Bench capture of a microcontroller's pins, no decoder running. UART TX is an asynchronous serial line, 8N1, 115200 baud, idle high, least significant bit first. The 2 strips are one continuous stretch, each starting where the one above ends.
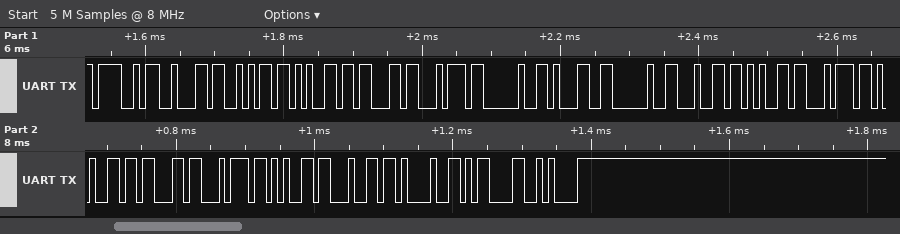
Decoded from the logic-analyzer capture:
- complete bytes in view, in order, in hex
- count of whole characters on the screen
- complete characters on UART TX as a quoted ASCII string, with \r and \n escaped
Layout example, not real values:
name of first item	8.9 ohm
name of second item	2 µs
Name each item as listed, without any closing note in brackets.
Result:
complete bytes in view, in order, in hex	4F 62 6A 65 63 74 20 31 20 64 65 74 65 63 74 65 64 21 0D 0A
count of whole characters on the screen	20
complete characters on UART TX as a quoted ASCII string, with \r and \n escaped	"Object 1 detected!\r\n"
